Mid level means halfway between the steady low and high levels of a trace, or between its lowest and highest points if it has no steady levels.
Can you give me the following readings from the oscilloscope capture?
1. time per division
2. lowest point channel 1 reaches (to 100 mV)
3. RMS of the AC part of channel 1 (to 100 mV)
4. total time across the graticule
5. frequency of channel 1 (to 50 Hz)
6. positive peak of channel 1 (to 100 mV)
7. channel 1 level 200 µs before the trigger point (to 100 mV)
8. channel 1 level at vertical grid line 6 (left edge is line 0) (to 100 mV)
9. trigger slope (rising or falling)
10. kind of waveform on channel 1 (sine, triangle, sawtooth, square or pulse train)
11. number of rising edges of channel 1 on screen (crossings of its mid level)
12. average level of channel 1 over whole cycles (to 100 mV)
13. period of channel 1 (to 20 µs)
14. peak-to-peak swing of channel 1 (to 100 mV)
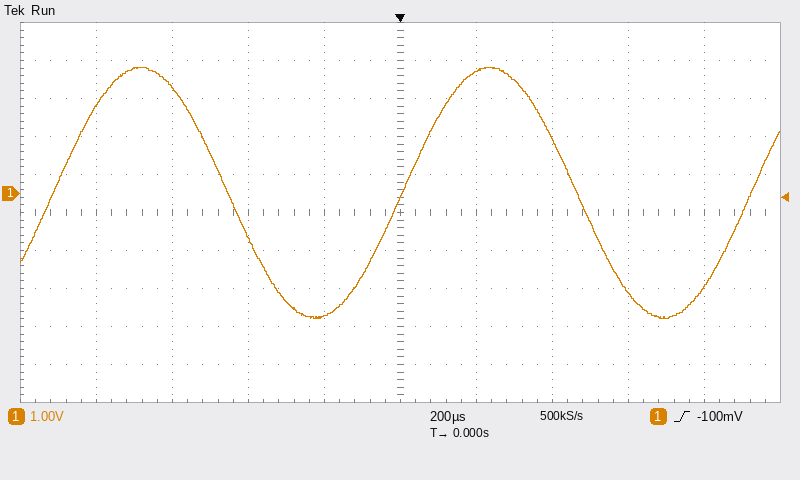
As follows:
200 µs
-3.3 V
2.3 V
2 ms
1.10 kHz
3.3 V
-3.2 V
3.2 V
rising
sine
3
0.0 V
920 µs
6.6 V
